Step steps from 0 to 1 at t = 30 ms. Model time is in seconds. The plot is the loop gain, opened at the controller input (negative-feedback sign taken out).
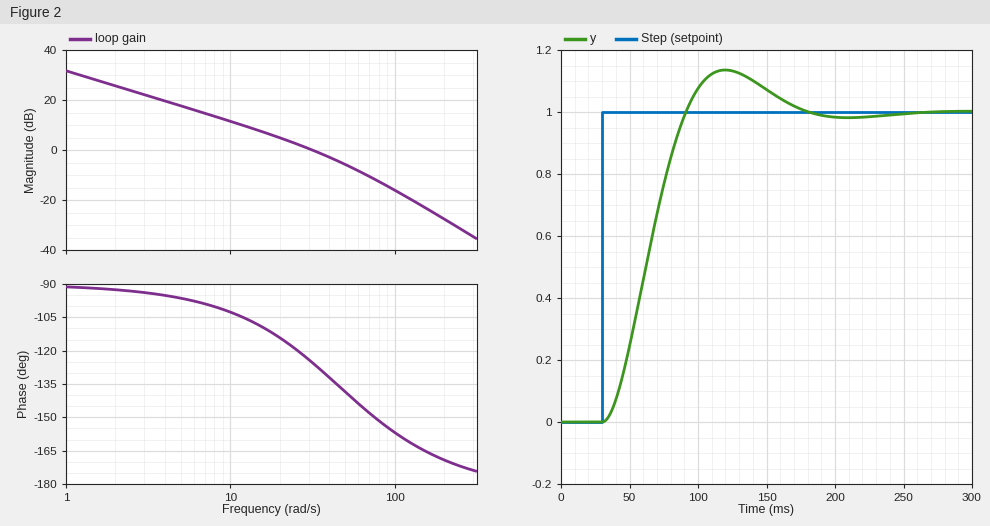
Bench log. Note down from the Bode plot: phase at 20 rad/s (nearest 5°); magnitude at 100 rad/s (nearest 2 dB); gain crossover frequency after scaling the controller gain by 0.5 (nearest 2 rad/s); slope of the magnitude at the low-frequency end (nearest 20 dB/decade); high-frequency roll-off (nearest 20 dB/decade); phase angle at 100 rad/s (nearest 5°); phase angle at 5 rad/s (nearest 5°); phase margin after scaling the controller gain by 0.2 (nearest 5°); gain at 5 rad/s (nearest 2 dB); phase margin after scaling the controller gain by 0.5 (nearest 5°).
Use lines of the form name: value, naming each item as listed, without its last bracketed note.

phase at 20 rad/s: -115°
magnitude at 100 rad/s: -16 dB
gain crossover frequency after scaling the controller gain by 0.5: 18 rad/s
slope of the magnitude at the low-frequency end: -20 dB/decade
high-frequency roll-off: -40 dB/decade
phase angle at 100 rad/s: -155°
phase angle at 5 rad/s: -95°
phase margin after scaling the controller gain by 0.2: 80°
gain at 5 rad/s: 18 dB
phase margin after scaling the controller gain by 0.5: 70°
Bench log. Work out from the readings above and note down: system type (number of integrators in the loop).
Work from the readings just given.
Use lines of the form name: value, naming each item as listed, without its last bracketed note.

system type: 1
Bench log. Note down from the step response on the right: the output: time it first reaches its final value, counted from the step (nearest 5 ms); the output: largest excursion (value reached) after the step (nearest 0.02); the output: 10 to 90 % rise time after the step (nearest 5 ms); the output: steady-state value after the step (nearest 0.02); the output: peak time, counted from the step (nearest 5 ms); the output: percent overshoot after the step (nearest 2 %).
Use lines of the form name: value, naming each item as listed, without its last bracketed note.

the output: time it first reaches its final value, counted from the step: 60 ms
the output: largest excursion (value reached) after the step: 1.14
the output: 10 to 90 % rise time after the step: 40 ms
the output: steady-state value after the step: 1.00
the output: peak time, counted from the step: 90 ms
the output: percent overshoot after the step: 14 %
